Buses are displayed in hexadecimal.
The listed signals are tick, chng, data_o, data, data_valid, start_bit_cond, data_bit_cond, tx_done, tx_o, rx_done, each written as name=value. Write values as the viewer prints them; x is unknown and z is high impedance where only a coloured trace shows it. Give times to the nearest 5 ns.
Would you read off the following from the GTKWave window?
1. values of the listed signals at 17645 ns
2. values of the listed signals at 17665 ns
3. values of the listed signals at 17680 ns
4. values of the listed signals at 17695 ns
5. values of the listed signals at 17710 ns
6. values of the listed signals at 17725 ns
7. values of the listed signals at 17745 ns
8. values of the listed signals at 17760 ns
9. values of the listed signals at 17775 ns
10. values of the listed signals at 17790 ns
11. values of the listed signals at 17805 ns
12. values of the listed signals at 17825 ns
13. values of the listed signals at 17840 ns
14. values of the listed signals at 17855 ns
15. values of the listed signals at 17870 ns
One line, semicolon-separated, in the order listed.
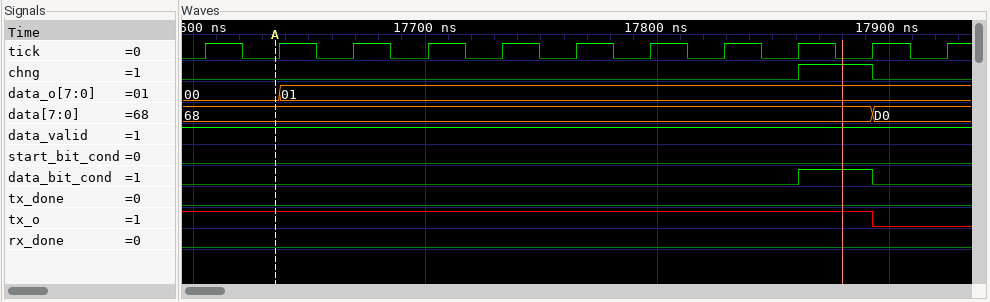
tick=1, chng=0, data_o=01, data=68, data_valid=1, start_bit_cond=0, data_bit_cond=0, tx_done=0, tx_o=1, rx_done=0; tick=0, chng=0, data_o=01, data=68, data_valid=1, start_bit_cond=0, data_bit_cond=0, tx_done=0, tx_o=1, rx_done=0; tick=1, chng=0, data_o=01, data=68, data_valid=1, start_bit_cond=0, data_bit_cond=0, tx_done=0, tx_o=1, rx_done=0; tick=0, chng=0, data_o=01, data=68, data_valid=1, start_bit_cond=0, data_bit_cond=0, tx_done=0, tx_o=1, rx_done=0; tick=1, chng=0, data_o=01, data=68, data_valid=1, start_bit_cond=0, data_bit_cond=0, tx_done=0, tx_o=1, rx_done=0; tick=0, chng=0, data_o=01, data=68, data_valid=1, start_bit_cond=0, data_bit_cond=0, tx_done=0, tx_o=1, rx_done=0; tick=1, chng=0, data_o=01, data=68, data_valid=1, start_bit_cond=0, data_bit_cond=0, tx_done=0, tx_o=1, rx_done=0; tick=0, chng=0, data_o=01, data=68, data_valid=1, start_bit_cond=0, data_bit_cond=0, tx_done=0, tx_o=1, rx_done=0; tick=1, chng=0, data_o=01, data=68, data_valid=1, start_bit_cond=0, data_bit_cond=0, tx_done=0, tx_o=1, rx_done=0; tick=0, chng=0, data_o=01, data=68, data_valid=1, start_bit_cond=0, data_bit_cond=0, tx_done=0, tx_o=1, rx_done=0; tick=1, chng=0, data_o=01, data=68, data_valid=1, start_bit_cond=0, data_bit_cond=0, tx_done=0, tx_o=1, rx_done=0; tick=0, chng=0, data_o=01, data=68, data_valid=1, start_bit_cond=0, data_bit_cond=0, tx_done=0, tx_o=1, rx_done=0; tick=1, chng=0, data_o=01, data=68, data_valid=1, start_bit_cond=0, data_bit_cond=0, tx_done=0, tx_o=1, rx_done=0; tick=0, chng=0, data_o=01, data=68, data_valid=1, start_bit_cond=0, data_bit_cond=0, tx_done=0, tx_o=1, rx_done=0; tick=1, chng=1, data_o=01, data=68, data_valid=1, start_bit_cond=0, data_bit_cond=1, tx_done=0, tx_o=1, rx_done=0
